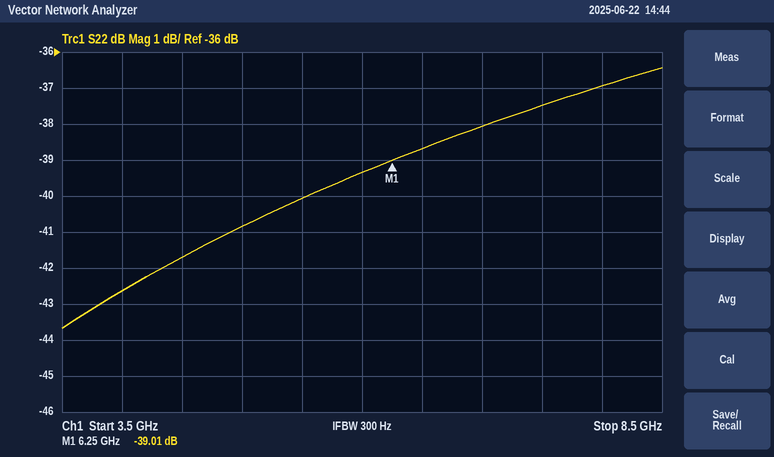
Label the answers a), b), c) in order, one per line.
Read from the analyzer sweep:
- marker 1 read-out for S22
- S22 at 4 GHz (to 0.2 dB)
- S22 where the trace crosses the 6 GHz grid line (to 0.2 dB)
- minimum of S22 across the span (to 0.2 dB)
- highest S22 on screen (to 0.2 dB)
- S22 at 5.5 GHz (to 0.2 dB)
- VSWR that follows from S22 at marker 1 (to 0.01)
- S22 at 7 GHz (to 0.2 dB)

a) -39.01 dB
b) -42.6 dB
c) -39.4 dB
d) -43.6 dB
e) -36.4 dB
f) -40.0 dB
g) 1.02
h) -38.0 dB
